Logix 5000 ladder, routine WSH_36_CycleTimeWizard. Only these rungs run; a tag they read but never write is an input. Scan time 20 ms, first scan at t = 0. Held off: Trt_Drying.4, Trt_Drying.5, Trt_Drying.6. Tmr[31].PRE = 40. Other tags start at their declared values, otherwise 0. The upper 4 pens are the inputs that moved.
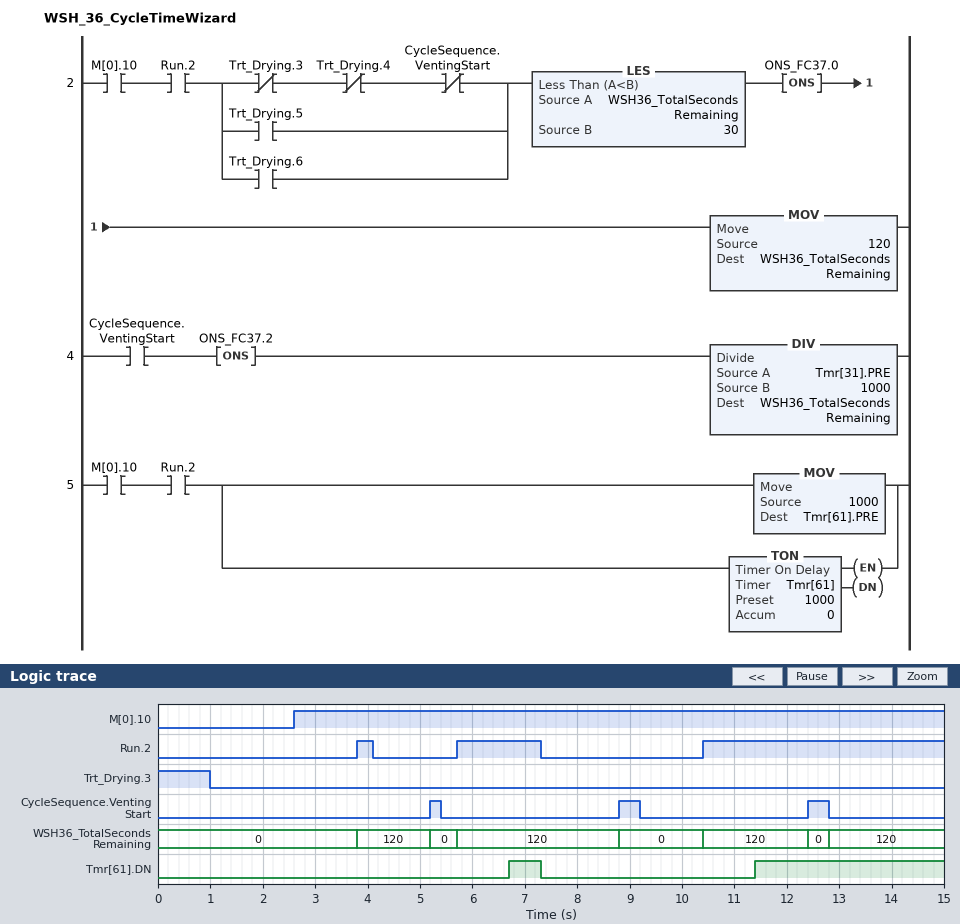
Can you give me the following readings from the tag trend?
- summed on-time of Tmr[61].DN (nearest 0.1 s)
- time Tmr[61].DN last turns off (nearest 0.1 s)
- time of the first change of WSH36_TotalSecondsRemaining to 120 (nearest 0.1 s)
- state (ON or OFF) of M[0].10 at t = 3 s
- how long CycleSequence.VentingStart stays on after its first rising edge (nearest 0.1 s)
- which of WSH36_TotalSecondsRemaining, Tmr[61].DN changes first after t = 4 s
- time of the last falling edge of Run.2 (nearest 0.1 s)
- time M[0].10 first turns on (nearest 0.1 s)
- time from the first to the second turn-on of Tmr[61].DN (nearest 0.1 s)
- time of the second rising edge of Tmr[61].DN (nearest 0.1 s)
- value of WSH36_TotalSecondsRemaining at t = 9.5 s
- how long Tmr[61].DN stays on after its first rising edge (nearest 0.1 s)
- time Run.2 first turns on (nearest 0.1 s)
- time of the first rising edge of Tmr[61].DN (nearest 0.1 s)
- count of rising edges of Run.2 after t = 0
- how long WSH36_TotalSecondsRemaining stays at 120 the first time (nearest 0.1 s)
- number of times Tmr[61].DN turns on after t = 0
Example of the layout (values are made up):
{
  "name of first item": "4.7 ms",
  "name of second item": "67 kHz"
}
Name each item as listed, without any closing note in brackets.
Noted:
{
  "summed on-time of Tmr[61].DN": "4.2 s",
  "time Tmr[61].DN last turns off": "7.3 s",
  "time of the first change of WSH36_TotalSecondsRemaining to 120": "3.8 s",
  "state (ON or OFF) of M[0].10 at t = 3 s": "ON",
  "how long CycleSequence.VentingStart stays on after its first rising edge": "0.2 s",
  "which of WSH36_TotalSecondsRemaining, Tmr[61].DN changes first after t = 4 s": "WSH36_TotalSecondsRemaining",
  "time of the last falling edge of Run.2": "7.3 s",
  "time M[0].10 first turns on": "2.6 s",
  "time from the first to the second turn-on of Tmr[61].DN": "4.7 s",
  "time of the second rising edge of Tmr[61].DN": "11.4 s",
  "value of WSH36_TotalSecondsRemaining at t = 9.5 s": "0",
  "how long Tmr[61].DN stays on after its first rising edge": "0.6 s",
  "time Run.2 first turns on": "3.8 s",
  "time of the first rising edge of Tmr[61].DN": "6.7 s",
  "count of rising edges of Run.2 after t = 0": "3",
  "how long WSH36_TotalSecondsRemaining stays at 120 the first time": "1.4 s",
  "number of times Tmr[61].DN turns on after t = 0": "2"
}
